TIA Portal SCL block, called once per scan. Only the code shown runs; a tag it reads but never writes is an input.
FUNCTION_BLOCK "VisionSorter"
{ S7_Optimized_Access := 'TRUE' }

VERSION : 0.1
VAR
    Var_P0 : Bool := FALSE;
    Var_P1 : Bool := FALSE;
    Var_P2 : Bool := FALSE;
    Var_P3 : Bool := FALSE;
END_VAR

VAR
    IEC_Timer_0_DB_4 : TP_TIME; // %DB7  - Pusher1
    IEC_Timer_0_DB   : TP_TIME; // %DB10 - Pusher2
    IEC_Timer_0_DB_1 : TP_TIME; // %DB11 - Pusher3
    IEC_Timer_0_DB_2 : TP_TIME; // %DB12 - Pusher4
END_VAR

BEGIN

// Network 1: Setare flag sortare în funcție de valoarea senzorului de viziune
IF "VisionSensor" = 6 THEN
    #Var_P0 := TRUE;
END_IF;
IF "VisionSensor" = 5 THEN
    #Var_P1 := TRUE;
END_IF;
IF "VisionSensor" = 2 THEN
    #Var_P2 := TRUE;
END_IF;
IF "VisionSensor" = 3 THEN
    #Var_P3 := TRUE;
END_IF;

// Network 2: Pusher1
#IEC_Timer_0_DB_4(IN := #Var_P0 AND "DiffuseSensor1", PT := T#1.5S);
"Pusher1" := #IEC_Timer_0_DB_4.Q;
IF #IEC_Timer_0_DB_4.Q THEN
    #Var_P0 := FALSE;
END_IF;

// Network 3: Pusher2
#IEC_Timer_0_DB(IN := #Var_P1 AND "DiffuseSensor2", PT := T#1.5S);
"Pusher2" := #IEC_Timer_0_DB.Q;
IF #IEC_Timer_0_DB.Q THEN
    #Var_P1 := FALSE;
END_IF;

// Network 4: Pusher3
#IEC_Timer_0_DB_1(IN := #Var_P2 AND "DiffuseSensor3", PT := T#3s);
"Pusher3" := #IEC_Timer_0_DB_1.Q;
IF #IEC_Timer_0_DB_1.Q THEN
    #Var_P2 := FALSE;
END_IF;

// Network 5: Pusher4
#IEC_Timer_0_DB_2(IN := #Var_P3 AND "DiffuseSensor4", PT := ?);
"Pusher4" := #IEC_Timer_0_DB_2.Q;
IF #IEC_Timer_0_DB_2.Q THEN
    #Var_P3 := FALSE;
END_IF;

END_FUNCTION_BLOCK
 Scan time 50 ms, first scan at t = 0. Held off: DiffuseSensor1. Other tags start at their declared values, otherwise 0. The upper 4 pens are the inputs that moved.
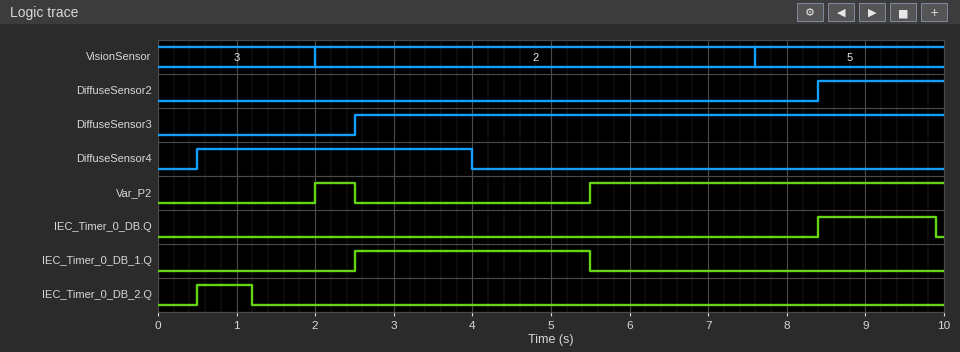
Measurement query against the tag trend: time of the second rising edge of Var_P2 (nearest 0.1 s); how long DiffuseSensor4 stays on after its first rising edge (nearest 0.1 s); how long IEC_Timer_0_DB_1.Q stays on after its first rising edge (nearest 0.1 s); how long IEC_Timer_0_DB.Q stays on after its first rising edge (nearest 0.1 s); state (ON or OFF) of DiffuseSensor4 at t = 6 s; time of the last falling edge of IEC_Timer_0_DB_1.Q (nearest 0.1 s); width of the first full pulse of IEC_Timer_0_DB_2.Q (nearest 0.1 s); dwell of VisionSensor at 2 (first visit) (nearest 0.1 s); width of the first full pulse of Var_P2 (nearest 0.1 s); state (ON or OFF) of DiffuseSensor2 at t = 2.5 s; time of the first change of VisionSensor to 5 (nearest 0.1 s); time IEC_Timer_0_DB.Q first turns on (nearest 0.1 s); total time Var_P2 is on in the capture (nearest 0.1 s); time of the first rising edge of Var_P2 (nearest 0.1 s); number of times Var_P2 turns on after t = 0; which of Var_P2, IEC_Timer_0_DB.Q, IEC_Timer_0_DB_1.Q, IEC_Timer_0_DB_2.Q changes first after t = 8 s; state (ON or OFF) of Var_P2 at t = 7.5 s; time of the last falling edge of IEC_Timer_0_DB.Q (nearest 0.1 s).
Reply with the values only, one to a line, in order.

5.5 s
3.5 s
3.0 s
1.5 s
OFF
5.5 s
0.7 s
5.6 s
0.5 s
OFF
7.6 s
8.4 s
5.0 s
2.0 s
2
IEC_Timer_0_DB.Q
ON
9.9 s
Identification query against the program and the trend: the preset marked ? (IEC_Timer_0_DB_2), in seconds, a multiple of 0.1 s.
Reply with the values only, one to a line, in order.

0.7 s
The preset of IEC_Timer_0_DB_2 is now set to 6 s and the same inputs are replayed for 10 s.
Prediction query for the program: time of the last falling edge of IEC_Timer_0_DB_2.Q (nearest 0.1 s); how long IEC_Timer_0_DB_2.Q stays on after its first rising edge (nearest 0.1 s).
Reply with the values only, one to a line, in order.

6.5 s
6.0 s
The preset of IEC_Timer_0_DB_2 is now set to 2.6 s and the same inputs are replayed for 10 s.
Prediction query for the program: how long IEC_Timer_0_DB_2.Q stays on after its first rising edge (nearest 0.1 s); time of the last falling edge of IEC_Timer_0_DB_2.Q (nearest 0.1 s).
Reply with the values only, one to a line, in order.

2.6 s
3.1 s
